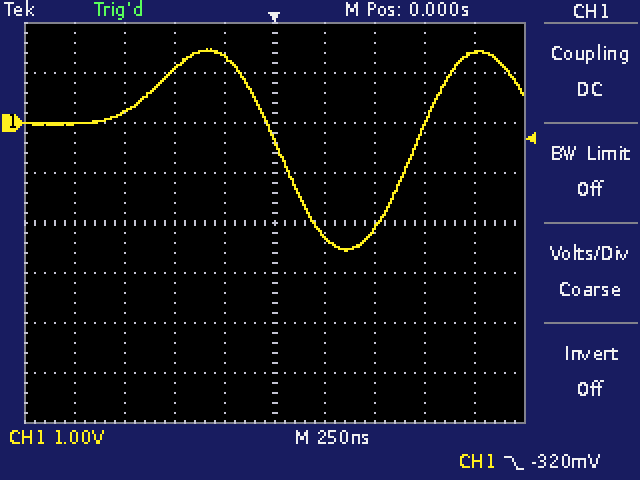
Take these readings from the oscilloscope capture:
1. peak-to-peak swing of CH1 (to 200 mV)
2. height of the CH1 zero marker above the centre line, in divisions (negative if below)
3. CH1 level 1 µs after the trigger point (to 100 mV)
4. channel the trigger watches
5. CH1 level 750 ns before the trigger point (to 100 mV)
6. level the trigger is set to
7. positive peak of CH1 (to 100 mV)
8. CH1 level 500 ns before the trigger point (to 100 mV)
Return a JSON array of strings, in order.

["4.0 V", "+2.0 div", "1.4 V", "CH1", "200 mV", "-320 mV", "1.5 V", "1.1 V"]
